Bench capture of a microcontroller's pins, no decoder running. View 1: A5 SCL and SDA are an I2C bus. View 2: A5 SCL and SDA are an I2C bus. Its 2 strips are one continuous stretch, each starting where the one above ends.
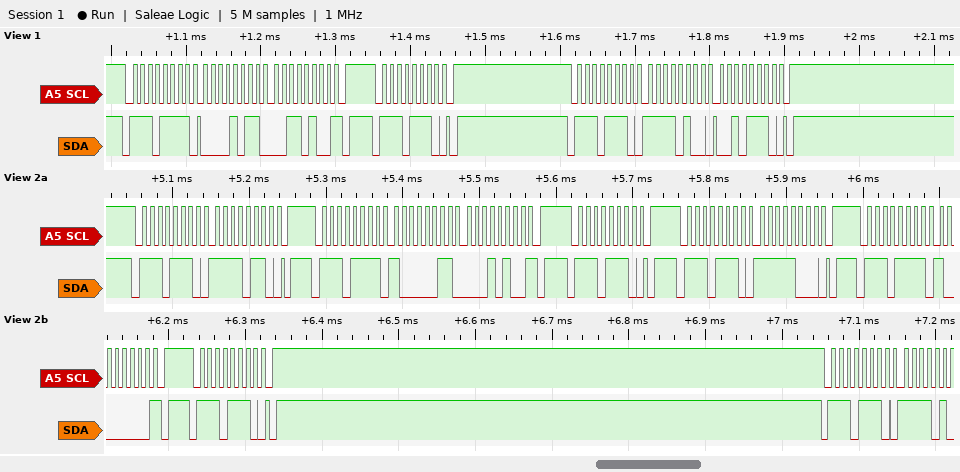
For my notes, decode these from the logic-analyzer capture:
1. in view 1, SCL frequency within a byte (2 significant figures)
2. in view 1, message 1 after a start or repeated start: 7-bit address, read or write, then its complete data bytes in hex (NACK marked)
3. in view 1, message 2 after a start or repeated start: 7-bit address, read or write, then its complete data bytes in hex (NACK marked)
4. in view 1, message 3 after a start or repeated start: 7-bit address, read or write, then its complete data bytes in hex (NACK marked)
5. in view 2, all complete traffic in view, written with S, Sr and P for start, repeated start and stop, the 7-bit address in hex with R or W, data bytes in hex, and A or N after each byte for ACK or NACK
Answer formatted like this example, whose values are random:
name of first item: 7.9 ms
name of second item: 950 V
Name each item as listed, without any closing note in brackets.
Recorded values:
in view 1, SCL frequency within a byte: 100 kHz
in view 1, message 1 after a start or repeated start: 7-bit address, read or write, then its complete data bytes in hex: 0x77 read: 0B 34 NACK
in view 1, message 2 after a start or repeated start: 7-bit address, read or write, then its complete data bytes in hex: 0x77 write
in view 1, message 3 after a start or repeated start: 7-bit address, read or write, then its complete data bytes in hex: 0x77 write: F4 2E
in view 2, all complete traffic in view, written with S, Sr and P for start, repeated start and stop, the 7-bit address in hex with R or W, data bytes in hex, and A or N after each byte for ACK or NACK: S 77W A F6 A P S 77R A 83 A 14 N P S 77W A P S 77W A F8 A P S 77R A 80 N P S 77W A P S 77W A
